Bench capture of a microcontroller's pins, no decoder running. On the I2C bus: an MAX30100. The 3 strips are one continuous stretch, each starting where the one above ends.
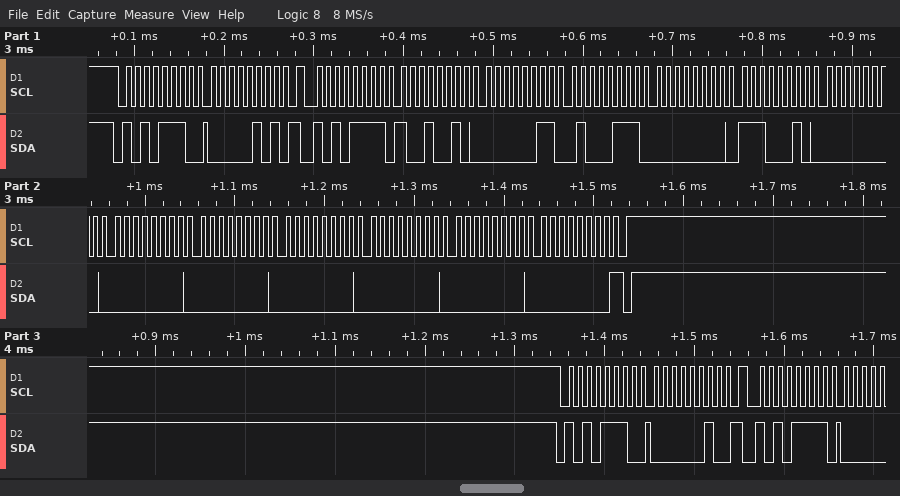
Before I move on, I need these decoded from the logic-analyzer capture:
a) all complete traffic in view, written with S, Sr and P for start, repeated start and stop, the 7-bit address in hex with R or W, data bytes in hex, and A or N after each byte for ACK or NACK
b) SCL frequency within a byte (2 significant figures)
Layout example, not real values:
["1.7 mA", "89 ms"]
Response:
["S 57W A 05 A Sr 57R A 92 A 03 A 47 A 00 A E2 A 00 A 00 A 00 A 00 A 00 A 00 A 00 N P S 57W A 02 A Sr 57R A", "100 kHz"]
